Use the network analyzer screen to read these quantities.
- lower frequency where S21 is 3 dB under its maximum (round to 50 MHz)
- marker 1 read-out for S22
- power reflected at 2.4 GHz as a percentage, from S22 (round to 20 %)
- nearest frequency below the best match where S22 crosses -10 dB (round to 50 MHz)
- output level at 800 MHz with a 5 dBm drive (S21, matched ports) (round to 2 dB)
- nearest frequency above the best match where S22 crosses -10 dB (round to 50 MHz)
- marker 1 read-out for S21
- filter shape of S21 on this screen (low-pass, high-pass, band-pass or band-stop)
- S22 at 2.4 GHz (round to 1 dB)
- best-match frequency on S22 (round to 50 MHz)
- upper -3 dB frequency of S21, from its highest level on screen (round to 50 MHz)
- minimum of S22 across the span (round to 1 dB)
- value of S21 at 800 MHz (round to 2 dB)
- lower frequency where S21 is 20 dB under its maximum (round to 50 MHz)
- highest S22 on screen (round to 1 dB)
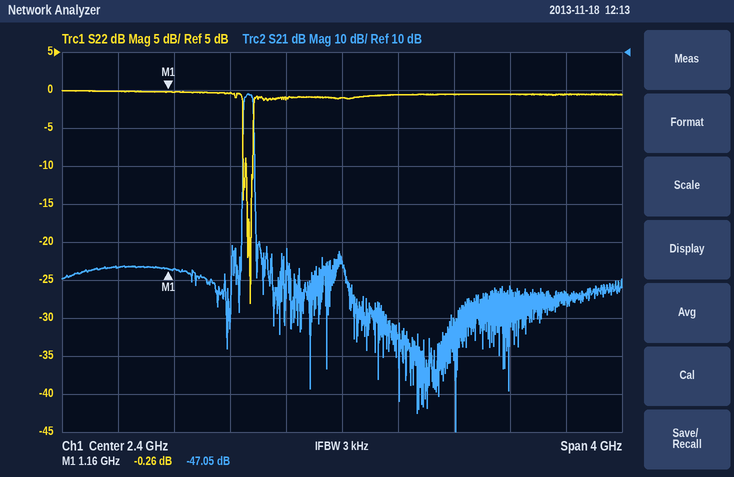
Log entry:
1.70 GHz
-0.26 dB
80 %
1.70 GHz
-42 dBm
1.75 GHz
-47.05 dB
band-pass
-1 dB
1.75 GHz
1.75 GHz
-28 dB
-46 dB
1.70 GHz
0 dB
